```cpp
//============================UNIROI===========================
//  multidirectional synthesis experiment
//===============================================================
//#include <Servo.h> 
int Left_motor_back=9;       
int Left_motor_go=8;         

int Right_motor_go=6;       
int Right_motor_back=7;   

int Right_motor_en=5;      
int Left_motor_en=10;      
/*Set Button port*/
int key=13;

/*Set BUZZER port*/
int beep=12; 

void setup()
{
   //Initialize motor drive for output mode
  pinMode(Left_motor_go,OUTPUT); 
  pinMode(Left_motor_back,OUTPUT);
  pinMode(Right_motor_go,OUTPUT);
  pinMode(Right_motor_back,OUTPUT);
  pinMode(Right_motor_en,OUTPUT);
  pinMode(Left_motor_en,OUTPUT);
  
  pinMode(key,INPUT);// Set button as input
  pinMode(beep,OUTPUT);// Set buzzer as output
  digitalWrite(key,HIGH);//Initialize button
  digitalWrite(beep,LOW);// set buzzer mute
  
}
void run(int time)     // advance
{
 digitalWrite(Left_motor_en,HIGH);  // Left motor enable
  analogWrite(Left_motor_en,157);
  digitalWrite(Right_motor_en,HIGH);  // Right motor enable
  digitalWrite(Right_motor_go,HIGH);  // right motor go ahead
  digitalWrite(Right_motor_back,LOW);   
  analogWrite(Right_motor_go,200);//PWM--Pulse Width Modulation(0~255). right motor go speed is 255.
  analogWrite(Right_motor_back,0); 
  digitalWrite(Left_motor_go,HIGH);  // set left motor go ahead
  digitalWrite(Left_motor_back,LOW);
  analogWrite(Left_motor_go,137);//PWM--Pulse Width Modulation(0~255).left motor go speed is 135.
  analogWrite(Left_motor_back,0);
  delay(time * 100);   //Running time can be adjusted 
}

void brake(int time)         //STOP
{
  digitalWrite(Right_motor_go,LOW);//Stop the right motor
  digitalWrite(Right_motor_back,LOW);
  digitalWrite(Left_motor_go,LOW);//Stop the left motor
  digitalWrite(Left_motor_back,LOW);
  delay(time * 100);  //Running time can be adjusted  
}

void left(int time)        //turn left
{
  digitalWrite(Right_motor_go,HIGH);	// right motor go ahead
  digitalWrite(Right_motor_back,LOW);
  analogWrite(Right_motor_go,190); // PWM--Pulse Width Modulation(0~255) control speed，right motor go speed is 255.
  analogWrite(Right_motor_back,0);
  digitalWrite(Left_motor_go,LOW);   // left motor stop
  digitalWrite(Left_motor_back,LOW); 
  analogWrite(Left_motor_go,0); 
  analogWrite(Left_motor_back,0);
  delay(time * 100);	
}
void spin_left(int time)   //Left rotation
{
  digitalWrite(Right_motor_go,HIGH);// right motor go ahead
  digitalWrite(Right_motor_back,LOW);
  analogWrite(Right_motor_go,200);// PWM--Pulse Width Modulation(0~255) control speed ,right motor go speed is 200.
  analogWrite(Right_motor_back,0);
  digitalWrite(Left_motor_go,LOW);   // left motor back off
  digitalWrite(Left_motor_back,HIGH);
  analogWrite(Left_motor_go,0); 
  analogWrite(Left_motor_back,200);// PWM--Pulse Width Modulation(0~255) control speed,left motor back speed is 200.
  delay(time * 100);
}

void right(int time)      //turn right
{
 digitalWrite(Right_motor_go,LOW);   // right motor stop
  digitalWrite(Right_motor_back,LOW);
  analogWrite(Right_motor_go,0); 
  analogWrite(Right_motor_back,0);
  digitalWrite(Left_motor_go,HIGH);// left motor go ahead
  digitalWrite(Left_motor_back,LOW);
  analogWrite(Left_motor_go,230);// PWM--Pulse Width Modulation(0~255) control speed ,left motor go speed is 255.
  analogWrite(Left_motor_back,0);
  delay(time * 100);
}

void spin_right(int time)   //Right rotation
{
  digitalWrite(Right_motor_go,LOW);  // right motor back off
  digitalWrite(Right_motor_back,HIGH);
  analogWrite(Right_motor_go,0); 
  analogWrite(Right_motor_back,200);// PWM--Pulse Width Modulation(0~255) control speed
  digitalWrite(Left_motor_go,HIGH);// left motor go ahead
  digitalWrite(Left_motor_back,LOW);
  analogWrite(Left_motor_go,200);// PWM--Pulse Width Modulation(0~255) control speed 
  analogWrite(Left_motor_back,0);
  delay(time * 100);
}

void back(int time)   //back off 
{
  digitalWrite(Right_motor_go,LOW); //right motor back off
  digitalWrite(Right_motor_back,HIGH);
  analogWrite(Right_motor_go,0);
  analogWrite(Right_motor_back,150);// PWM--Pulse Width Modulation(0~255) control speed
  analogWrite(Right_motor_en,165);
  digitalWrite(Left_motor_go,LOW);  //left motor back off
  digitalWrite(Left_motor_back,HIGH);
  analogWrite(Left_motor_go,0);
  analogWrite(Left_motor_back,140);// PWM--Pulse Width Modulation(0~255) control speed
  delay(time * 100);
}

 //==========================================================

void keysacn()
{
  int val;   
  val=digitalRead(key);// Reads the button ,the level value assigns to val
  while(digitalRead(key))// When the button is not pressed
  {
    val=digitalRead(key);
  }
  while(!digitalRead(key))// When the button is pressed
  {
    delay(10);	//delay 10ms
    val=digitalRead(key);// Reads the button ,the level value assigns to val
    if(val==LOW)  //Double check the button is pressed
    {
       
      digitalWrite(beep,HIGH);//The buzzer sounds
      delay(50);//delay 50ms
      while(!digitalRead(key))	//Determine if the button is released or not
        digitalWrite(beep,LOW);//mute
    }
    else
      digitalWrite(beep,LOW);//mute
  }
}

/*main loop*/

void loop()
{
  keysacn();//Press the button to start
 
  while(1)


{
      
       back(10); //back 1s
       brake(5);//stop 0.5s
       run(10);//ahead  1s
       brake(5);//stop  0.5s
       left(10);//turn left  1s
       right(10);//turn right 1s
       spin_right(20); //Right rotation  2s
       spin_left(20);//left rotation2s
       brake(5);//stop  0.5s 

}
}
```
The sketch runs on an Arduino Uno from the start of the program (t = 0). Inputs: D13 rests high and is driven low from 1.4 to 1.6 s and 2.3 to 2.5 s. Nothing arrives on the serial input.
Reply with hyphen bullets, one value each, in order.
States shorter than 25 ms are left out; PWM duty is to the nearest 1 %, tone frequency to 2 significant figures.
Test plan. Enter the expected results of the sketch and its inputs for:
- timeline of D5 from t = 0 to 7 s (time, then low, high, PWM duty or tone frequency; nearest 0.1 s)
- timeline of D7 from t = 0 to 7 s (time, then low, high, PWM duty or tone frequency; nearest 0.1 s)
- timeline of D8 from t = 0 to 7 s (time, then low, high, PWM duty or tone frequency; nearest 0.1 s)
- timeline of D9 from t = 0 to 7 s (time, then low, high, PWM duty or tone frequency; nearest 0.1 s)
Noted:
- 0 s low; 1.6 s PWM 65 %; 3.1 s high
- 0 s low; 1.6 s high; 2.6 s low; 6.6 s high
- 0 s low; 3.1 s high; 4.1 s low; 5.6 s high
- 0 s low; 1.6 s PWM 55 %; 2.6 s low
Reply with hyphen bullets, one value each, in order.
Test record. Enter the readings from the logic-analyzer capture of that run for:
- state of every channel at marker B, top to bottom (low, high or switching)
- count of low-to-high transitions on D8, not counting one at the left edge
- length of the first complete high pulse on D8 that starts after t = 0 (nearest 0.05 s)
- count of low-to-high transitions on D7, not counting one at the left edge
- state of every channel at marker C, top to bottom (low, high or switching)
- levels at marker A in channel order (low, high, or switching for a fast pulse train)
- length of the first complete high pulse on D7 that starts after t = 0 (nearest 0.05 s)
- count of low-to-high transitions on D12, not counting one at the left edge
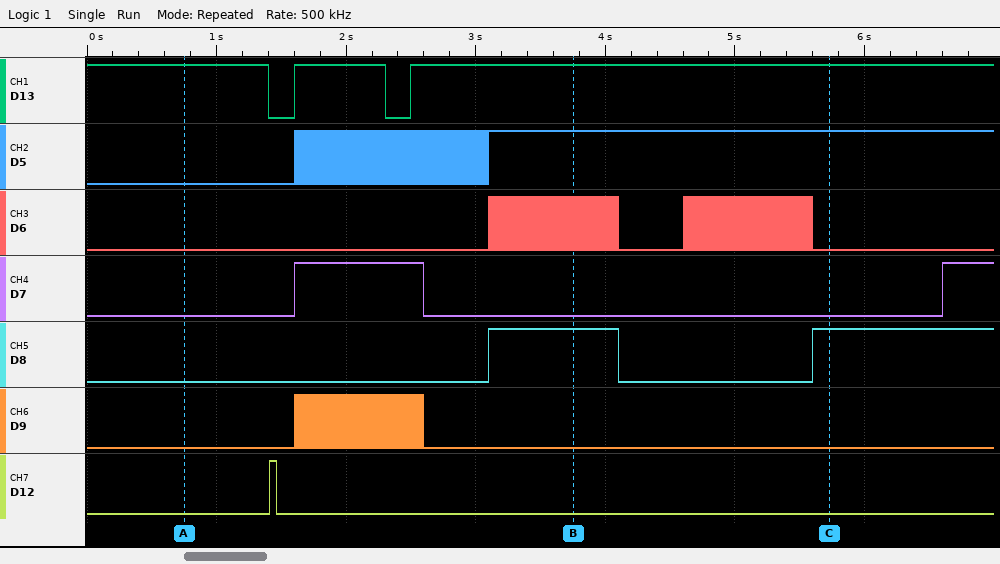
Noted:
- D13 high, D5 high, D6 switching, D7 low, D8 high, D9 low, D12 low
- 2
- 1.00 s
- 2
- D13 high, D5 high, D6 low, D7 low, D8 high, D9 low, D12 low
- D13 high, D5 low, D6 low, D7 low, D8 low, D9 low, D12 low
- 1.00 s
- 1
